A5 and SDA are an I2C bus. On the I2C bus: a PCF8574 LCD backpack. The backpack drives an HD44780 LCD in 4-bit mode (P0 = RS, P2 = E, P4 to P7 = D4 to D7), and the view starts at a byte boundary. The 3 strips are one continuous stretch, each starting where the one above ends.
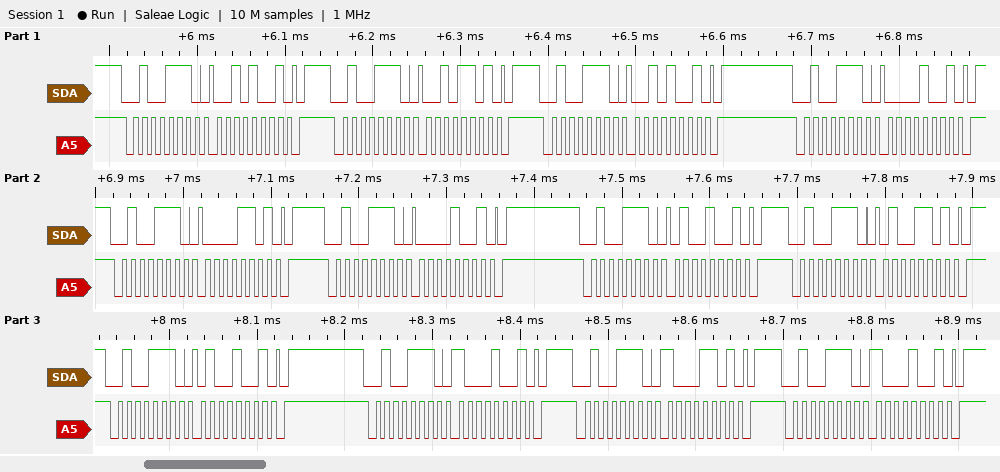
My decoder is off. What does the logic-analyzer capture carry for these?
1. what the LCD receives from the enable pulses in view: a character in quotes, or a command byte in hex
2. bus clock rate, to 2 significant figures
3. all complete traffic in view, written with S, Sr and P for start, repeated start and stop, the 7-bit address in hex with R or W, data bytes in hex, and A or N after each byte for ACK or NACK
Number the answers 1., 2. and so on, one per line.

1. ' ' 'H'
2. 100 kHz
3. S 27W A 29 A P S 27W A 2D A P S 27W A 29 A P S 27W A 09 A P S 27W A 0D A P S 27W A 09 A P S 27W A 49 A P S 27W A 4D A P S 27W A 49 A P S 27W A 89 A P S 27W A 8D A P S 27W A 89 A P
